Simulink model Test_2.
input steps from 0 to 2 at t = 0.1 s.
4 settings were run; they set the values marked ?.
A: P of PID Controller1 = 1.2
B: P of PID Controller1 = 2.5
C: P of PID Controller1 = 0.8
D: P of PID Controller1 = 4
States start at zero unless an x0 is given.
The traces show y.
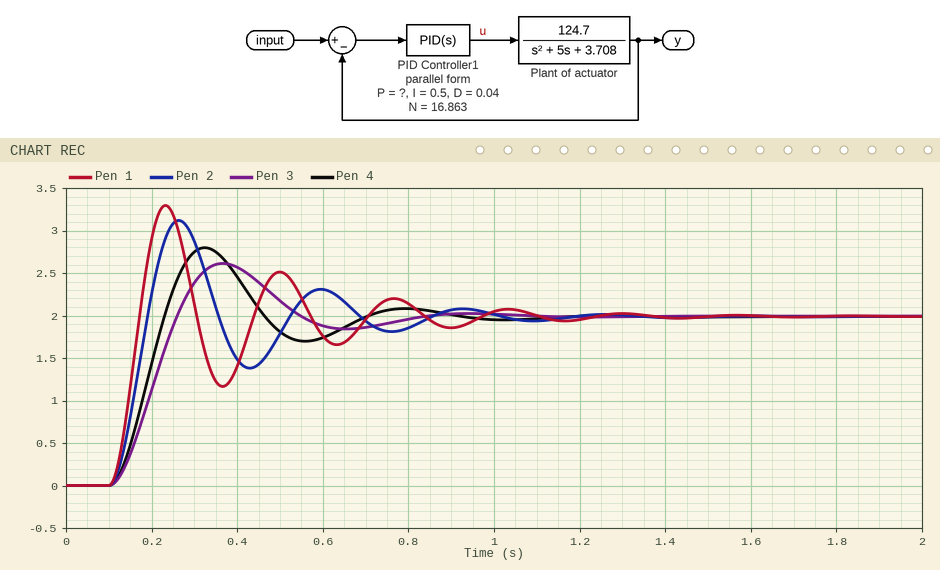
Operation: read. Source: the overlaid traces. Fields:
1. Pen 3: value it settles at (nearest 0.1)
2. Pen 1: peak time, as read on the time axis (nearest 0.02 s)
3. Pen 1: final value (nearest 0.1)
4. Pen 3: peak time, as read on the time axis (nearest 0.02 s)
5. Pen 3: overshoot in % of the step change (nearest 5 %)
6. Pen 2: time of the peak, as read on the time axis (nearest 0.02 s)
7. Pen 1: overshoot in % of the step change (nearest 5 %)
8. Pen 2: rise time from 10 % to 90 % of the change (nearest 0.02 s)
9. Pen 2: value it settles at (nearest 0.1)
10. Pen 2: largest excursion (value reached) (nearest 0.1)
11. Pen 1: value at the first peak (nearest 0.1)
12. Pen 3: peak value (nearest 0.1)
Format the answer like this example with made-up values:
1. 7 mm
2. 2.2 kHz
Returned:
1. 2.0
2. 0.24 s
3. 2.0
4. 0.36 s
5. 30 %
6. 0.26 s
7. 65 %
8. 0.06 s
9. 2.0
10. 3.1
11. 3.3
12. 2.6
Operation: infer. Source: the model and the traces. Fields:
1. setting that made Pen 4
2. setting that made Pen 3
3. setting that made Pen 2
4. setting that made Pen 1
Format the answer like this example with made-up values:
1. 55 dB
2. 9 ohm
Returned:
1. A
2. C
3. B
4. D
